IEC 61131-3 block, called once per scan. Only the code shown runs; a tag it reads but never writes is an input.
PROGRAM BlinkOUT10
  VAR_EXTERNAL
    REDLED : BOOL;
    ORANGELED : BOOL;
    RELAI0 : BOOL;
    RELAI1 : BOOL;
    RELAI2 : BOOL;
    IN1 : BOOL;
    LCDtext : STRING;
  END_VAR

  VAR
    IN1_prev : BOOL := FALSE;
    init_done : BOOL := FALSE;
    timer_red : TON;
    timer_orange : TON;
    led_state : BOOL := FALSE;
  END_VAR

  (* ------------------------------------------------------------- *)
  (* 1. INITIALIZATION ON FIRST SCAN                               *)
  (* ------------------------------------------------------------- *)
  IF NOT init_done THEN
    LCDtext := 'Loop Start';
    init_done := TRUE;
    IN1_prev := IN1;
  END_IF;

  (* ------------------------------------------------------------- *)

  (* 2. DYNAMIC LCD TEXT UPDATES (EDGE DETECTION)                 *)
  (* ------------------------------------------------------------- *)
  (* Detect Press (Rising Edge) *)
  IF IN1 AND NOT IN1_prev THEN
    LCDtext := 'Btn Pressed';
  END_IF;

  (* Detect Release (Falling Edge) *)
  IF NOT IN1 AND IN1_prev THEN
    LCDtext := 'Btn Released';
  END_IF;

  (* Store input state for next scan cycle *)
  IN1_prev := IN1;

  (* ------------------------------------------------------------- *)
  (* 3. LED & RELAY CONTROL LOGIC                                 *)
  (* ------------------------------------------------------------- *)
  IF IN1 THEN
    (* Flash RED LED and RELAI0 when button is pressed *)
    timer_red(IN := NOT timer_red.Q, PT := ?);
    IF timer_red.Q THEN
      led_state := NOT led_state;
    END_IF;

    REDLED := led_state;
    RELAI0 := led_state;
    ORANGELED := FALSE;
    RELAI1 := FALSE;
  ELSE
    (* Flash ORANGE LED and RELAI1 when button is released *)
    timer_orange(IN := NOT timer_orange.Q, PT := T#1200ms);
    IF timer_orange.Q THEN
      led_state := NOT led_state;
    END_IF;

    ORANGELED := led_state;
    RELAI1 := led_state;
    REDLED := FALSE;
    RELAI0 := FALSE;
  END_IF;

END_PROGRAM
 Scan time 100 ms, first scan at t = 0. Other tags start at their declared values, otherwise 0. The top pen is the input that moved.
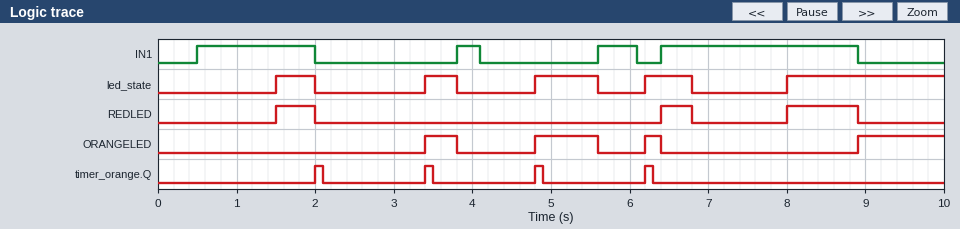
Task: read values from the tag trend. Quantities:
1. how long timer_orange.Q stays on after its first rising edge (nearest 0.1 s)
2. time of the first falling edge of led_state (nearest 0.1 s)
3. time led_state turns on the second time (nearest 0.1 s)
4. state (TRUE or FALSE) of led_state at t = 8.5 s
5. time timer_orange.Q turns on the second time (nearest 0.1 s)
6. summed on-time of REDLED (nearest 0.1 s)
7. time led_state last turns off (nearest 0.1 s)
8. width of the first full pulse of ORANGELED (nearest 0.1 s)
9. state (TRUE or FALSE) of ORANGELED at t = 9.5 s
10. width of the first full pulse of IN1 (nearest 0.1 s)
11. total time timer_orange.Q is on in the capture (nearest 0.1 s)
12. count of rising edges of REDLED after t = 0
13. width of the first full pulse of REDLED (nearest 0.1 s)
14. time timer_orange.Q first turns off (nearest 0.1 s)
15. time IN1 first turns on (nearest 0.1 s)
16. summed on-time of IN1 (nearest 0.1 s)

0.1 s
2.0 s
3.4 s
TRUE
3.4 s
1.8 s
6.8 s
0.4 s
TRUE
1.5 s
0.4 s
3
0.5 s
2.1 s
0.5 s
4.8 s
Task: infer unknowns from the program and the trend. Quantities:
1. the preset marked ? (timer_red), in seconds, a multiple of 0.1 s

1.0 s
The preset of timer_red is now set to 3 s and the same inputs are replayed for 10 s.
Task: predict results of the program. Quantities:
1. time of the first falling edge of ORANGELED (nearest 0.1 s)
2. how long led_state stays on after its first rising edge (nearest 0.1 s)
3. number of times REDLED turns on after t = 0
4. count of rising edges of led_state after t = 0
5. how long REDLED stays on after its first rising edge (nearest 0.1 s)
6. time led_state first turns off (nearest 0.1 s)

3.4 s
1.4 s
2
3
0.3 s
3.4 s
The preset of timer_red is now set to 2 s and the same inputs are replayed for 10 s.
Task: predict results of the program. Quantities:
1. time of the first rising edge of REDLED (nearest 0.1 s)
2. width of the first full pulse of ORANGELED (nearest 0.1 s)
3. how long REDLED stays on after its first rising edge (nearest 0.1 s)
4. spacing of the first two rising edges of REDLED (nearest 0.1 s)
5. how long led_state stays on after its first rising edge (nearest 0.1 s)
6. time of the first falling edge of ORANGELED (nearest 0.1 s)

3.8 s
1.4 s
0.3 s
2.2 s
1.4 s
3.4 s
